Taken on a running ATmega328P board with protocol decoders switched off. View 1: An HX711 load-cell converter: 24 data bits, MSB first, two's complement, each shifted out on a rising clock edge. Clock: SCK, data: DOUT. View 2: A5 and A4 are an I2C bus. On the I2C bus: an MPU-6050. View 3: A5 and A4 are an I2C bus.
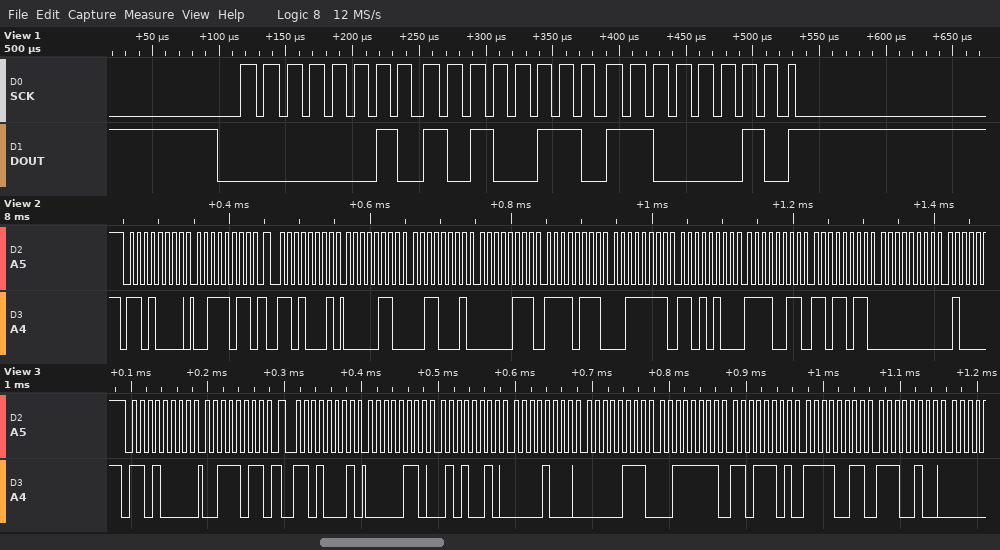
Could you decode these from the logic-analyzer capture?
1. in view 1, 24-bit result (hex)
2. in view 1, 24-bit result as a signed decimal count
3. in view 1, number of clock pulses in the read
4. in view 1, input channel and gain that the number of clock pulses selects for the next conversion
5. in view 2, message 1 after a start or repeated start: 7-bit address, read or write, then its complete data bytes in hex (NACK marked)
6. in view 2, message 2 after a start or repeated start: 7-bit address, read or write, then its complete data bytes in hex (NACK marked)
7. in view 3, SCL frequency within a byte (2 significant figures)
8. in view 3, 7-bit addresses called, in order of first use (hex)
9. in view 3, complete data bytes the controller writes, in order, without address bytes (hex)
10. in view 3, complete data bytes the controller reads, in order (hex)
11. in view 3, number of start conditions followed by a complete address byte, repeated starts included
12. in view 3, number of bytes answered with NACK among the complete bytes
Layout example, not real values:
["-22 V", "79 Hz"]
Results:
["0x02A6C2", "173762", "25", "channel A, gain 128", "0x68 write: 3B", "0x68 read: 06 31 07 F7 3F D4 F3 DB 00", "100 kHz", "0x68", "3B", "06 52 08 07 3F DD F3 E4", "2", "0"]
